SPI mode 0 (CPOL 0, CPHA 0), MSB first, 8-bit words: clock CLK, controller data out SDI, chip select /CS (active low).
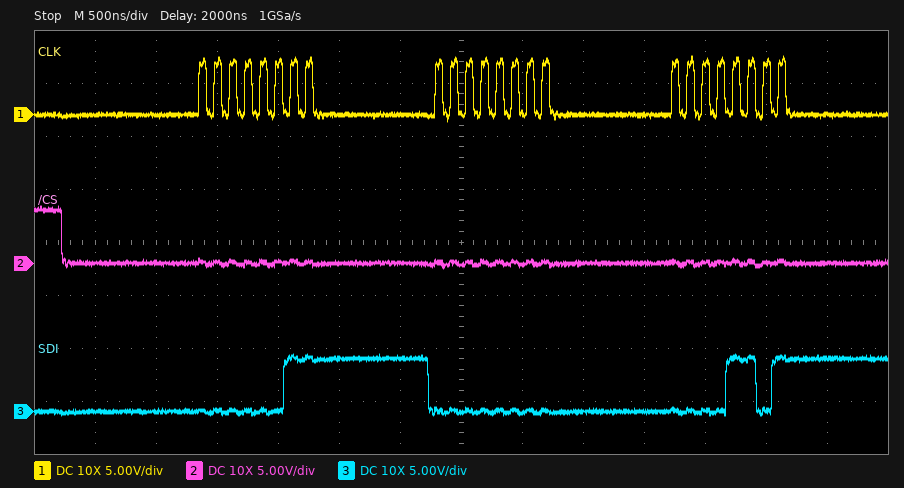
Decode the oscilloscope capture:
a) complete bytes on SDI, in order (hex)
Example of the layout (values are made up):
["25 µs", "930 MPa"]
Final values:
["03 00 0D"]
